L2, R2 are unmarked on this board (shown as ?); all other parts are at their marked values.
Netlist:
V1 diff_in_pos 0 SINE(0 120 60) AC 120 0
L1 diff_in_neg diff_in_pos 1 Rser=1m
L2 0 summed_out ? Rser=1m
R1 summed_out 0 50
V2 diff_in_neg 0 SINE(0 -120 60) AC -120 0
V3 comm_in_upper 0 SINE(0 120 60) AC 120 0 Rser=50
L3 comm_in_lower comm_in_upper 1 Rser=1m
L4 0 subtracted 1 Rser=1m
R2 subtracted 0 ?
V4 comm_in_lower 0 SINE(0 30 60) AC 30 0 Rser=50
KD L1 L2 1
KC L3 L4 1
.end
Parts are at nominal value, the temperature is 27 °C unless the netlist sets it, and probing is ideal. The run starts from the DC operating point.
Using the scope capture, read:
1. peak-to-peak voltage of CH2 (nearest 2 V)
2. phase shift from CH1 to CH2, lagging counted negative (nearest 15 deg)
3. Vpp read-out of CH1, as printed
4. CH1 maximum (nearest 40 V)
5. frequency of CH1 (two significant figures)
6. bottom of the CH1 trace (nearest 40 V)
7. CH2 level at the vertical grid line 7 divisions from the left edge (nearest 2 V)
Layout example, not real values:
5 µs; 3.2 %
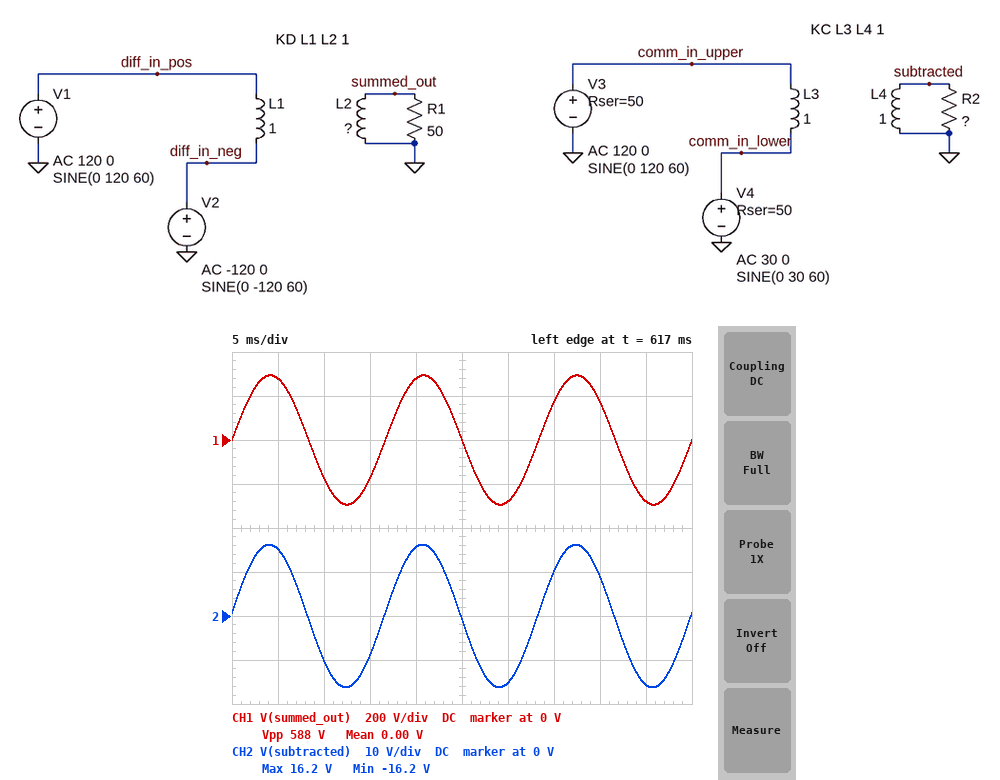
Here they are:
32 V; 0 deg; 588 V; 280 V; 60 Hz; -280 V; 10 V
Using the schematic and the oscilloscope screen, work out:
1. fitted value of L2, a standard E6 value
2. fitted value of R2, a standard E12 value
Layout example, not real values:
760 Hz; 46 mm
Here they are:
1.5 H; 22 Ω
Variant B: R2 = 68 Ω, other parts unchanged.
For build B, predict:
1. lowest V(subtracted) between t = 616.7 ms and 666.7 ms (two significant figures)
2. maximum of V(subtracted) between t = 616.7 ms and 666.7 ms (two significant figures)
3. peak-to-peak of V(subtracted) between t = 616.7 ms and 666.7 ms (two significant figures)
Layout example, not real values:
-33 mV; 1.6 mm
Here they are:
-36 V; 36 V; 72 V
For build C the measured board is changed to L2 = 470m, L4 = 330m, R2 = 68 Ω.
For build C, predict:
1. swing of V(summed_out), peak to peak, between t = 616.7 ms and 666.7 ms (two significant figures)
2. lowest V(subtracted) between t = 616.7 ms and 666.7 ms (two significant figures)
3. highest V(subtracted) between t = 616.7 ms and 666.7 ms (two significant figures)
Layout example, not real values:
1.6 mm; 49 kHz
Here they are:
330 V; -34 V; 34 V
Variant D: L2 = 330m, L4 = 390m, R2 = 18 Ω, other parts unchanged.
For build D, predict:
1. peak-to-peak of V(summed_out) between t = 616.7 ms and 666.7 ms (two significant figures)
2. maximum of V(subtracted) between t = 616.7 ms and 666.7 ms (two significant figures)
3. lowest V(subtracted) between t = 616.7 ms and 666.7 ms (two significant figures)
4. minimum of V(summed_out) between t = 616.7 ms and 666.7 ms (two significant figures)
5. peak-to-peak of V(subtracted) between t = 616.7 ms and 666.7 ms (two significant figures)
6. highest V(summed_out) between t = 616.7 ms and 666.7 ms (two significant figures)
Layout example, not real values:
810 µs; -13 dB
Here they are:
280 V; 18 V; -18 V; -140 V; 35 V; 140 V
